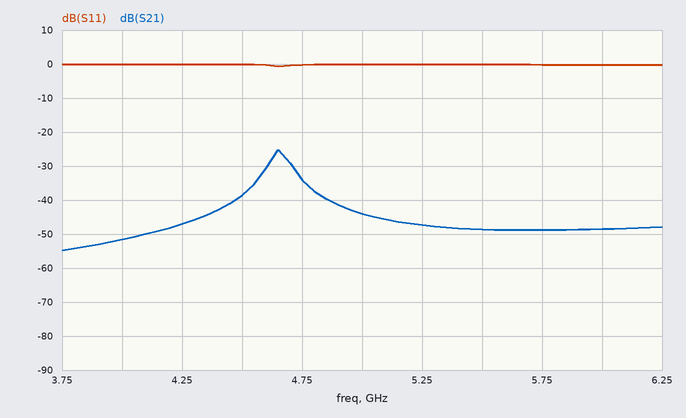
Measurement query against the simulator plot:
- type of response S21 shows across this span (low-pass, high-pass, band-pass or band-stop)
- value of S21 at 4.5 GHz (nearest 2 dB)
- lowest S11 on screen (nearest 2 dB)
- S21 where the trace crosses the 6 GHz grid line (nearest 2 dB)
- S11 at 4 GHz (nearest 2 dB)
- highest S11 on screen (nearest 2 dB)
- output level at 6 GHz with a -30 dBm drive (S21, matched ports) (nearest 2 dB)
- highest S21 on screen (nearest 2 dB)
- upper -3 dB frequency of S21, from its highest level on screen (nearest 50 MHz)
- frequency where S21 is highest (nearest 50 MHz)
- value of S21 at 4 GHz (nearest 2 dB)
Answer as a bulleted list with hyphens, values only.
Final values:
- band-pass
- -38 dB
- 0 dB
- -48 dB
- 0 dB
- 0 dB
- -78 dBm
- -26 dB
- 4.70 GHz
- 4.65 GHz
- -52 dB
